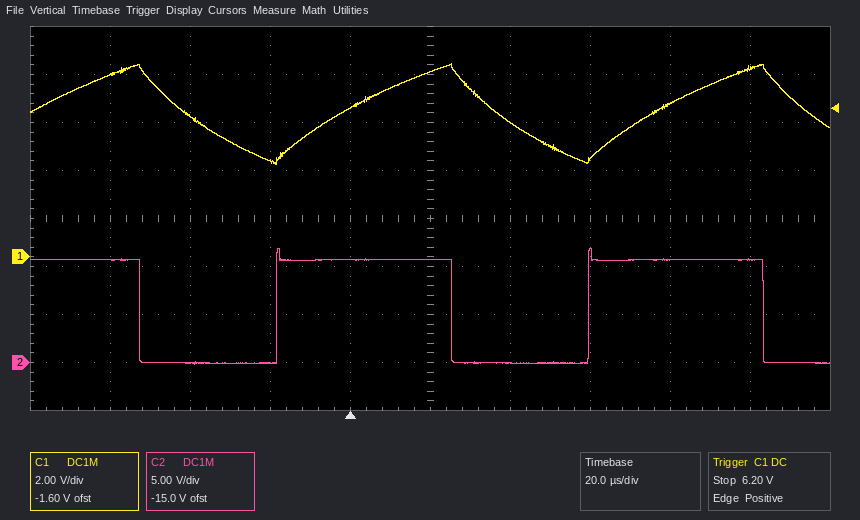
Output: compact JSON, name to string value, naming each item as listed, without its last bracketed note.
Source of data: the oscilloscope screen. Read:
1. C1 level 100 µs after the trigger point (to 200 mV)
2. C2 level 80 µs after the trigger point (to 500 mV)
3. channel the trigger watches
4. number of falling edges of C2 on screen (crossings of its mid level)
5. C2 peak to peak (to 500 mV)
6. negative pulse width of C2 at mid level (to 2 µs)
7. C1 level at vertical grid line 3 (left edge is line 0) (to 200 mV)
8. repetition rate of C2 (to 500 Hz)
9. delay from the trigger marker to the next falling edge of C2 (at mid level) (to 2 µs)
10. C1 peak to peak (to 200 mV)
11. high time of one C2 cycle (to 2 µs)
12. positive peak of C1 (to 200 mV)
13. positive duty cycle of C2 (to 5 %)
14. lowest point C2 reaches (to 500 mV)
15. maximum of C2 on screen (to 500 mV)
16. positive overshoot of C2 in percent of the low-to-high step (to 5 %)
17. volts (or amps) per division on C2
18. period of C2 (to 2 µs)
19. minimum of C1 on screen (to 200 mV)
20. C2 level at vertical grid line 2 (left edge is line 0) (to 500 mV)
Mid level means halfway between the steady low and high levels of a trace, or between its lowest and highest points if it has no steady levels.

{"C1 level 100 µs after the trigger point": "7.8 V", "C2 level 80 µs after the trigger point": "10.5 V", "channel the trigger watches": "C1", "number of falling edges of C2 on screen": "3", "C2 peak to peak": "12.0 V", "negative pulse width of C2 at mid level": "34 µs", "C1 level at vertical grid line 3 (left edge is line 0)": "4.0 V", "repetition rate of C2": "13.0 kHz", "delay from the trigger marker to the next falling edge of C2 (at mid level)": "26 µs", "C1 peak to peak": "4.2 V", "high time of one C2 cycle": "44 µs", "positive peak of C1": "8.0 V", "positive duty cycle of C2": "55 %", "lowest point C2 reaches": "0.0 V", "maximum of C2 on screen": "12.0 V", "positive overshoot of C2 in percent of the low-to-high step": "10 %", "volts (or amps) per division on C2": "5 V", "period of C2": "78 µs", "minimum of C1 on screen": "3.8 V", "C2 level at vertical grid line 2 (left edge is line 0)": "0.0 V"}
